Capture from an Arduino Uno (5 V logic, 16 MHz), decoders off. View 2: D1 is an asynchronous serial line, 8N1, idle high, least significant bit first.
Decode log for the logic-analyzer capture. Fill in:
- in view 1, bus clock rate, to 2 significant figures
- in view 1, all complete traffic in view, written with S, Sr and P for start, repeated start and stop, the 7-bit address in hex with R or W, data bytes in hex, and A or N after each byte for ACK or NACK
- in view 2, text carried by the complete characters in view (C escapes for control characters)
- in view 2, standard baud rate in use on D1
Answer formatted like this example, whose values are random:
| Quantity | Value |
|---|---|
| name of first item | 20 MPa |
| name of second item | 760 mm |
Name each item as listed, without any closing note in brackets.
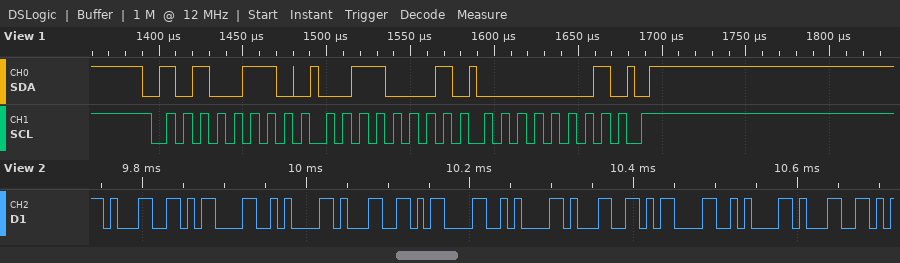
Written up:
| Quantity | Value |
|---|---|
| in view 1, bus clock rate, to 2 significant figures | 100 kHz |
| in view 1, all complete traffic in view, written with S, Sr and P for start, repeated start and stop, the 7-bit address in hex with R or W, data bytes in hex, and A or N after each byte for ACK or NACK | S 53W A 31 A 01 A P |
| in view 2, text carried by the complete characters in view | "1\r\n1\r\n1\r\n1" |
| in view 2, standard baud rate in use on D1 | 115200 baud |
